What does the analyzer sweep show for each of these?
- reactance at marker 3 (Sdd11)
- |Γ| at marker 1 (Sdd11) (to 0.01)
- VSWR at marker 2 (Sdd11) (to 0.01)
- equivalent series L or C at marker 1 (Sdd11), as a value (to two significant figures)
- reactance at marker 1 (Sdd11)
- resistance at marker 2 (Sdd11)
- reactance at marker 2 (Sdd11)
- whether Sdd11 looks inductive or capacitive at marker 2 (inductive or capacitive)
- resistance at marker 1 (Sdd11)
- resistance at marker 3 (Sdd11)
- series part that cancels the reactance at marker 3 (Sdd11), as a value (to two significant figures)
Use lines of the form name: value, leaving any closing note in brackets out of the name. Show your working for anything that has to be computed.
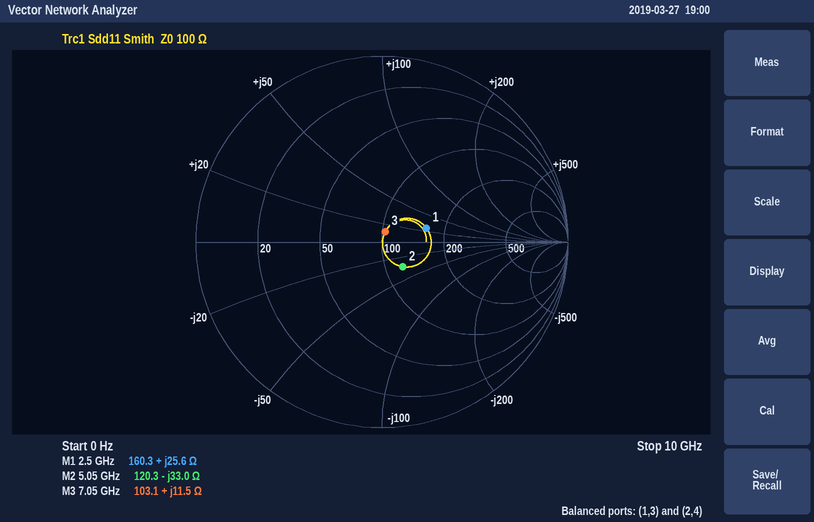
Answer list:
reactance at marker 3: +11.5 Ω
|Γ| at marker 1 (Sdd11): 0.25
VSWR at marker 2 (Sdd11): 1.42
equivalent series L or C at marker 1 (Sdd11), as a value: L = 25.6 Ω/(2π × 2.5 GHz) ≈ 1.6 nH
reactance at marker 1: +25.6 Ω
resistance at marker 2: 120.3 Ω
reactance at marker 2: -33.0 Ω
whether Sdd11 looks inductive or capacitive at marker 2: capacitive
resistance at marker 1: 160.3 Ω
resistance at marker 3: 103.1 Ω
series part that cancels the reactance at marker 3 (Sdd11), as a value: C = 1/(2π × 7.05 GHz × 11.5 Ω) ≈ 2.0 pF
